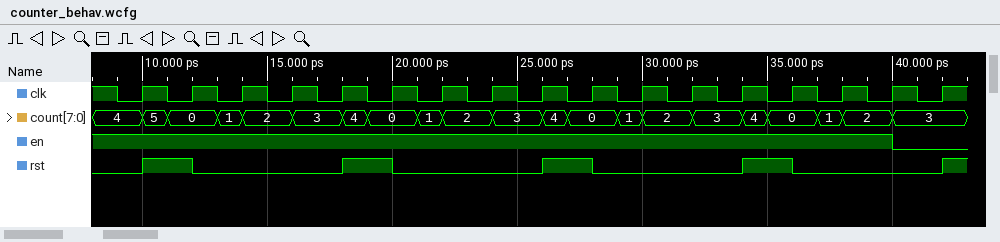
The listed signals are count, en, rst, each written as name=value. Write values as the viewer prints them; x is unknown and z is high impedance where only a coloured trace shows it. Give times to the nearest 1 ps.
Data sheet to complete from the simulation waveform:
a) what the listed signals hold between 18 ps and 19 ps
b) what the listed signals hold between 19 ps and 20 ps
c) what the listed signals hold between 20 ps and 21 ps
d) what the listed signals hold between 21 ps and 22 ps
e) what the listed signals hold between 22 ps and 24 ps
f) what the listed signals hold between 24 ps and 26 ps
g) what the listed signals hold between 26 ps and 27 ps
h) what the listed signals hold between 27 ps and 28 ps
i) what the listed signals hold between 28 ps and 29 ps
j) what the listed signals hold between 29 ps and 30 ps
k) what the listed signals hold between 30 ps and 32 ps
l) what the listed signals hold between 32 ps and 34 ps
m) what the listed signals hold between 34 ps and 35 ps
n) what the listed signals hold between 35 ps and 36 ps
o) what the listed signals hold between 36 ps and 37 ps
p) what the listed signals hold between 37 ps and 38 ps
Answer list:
count=4, en=1, rst=1
count=0, en=1, rst=1
count=0, en=1, rst=0
count=1, en=1, rst=0
count=2, en=1, rst=0
count=3, en=1, rst=0
count=4, en=1, rst=1
count=0, en=1, rst=1
count=0, en=1, rst=0
count=1, en=1, rst=0
count=2, en=1, rst=0
count=3, en=1, rst=0
count=4, en=1, rst=1
count=0, en=1, rst=1
count=0, en=1, rst=0
count=1, en=1, rst=0
